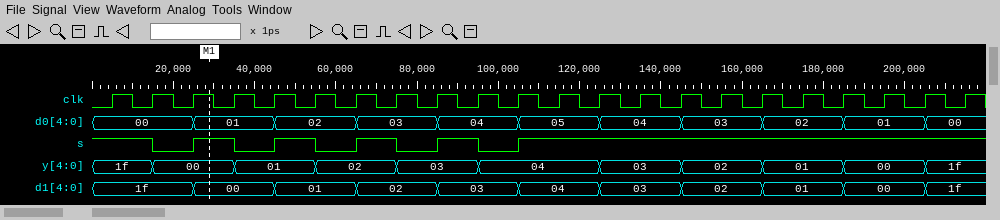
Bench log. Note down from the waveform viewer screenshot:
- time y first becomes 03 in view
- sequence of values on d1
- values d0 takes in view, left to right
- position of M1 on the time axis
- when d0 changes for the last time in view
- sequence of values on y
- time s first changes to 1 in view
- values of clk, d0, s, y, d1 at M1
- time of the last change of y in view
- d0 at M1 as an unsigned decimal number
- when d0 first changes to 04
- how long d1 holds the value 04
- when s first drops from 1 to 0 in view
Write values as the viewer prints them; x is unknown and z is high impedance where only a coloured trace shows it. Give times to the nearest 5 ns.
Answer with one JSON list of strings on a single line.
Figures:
["75 ns", "1f, 00, 01, 02, 03, 04, 03, 02, 01, 00, 1f", "00, 01, 02, 03, 04, 05, 04, 03, 02, 01, 00", "30 ns", "205 ns", "1f, 00, 01, 02, 03, 04, 03, 02, 01, 00, 1f", "25 ns", "clk=1, d0=01, s=1, y=00, d1=00", "205 ns", "1", "85 ns", "20 ns", "15 ns"]
